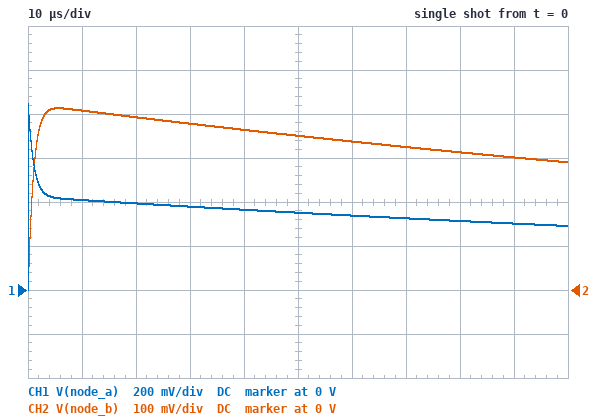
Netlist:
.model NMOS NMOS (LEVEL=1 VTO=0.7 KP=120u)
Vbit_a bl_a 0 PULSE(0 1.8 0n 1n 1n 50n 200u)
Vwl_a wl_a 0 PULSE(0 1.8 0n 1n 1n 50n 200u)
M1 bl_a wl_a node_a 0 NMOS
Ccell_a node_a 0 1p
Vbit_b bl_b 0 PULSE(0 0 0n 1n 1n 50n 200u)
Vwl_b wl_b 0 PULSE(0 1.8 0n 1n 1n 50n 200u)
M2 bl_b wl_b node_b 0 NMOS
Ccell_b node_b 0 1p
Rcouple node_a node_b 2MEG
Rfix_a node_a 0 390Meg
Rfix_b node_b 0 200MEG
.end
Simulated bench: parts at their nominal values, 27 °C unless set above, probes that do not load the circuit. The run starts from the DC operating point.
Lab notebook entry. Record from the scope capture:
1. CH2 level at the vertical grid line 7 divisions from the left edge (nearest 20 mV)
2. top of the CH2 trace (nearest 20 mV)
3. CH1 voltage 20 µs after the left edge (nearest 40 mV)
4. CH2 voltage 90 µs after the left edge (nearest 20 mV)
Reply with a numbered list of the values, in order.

1. 320 mV
2. 420 mV
3. 400 mV
4. 300 mV
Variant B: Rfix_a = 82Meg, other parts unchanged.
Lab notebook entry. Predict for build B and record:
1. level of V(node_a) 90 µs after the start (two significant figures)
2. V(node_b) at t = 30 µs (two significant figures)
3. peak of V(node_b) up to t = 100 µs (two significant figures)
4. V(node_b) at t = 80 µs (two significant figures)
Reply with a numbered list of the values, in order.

1. 190 mV
2. 330 mV
3. 400 mV
4. 210 mV
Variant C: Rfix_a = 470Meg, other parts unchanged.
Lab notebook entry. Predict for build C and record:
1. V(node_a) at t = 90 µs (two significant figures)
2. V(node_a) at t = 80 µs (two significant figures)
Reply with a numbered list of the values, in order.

1. 310 mV
2. 320 mV
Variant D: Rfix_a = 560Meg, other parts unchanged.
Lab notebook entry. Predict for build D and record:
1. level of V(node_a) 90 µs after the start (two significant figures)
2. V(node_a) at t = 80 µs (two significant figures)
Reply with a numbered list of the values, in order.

1. 310 mV
2. 320 mV
